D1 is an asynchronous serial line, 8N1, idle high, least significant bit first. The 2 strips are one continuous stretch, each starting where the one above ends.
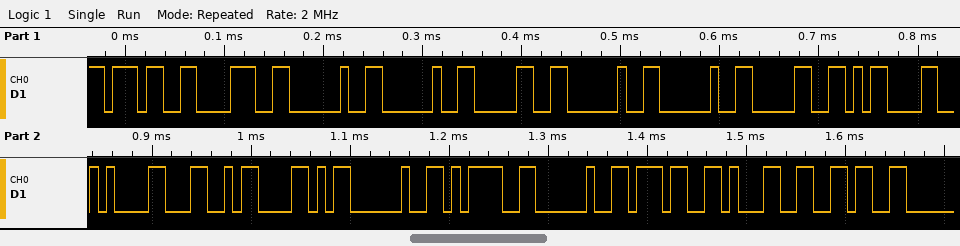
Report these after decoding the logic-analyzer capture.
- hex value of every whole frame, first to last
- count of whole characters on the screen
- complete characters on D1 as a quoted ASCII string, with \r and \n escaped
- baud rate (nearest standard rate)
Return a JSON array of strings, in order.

["0x37 0x38 0x20 0x20 0x30 0x20 0x20 0x30 0x0D 0x0A 0x4C 0x58 0x20 0x3D 0x20 0x37 0x31 0x36", "18", "\"78  0  0\\r\\nLX = 716\"", "115200 baud"]
